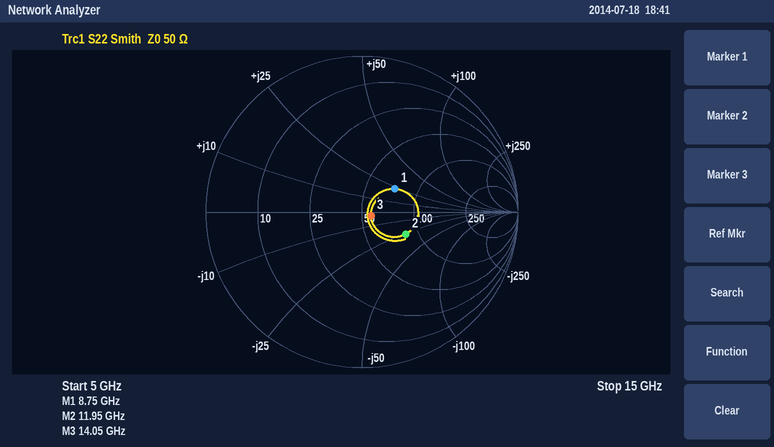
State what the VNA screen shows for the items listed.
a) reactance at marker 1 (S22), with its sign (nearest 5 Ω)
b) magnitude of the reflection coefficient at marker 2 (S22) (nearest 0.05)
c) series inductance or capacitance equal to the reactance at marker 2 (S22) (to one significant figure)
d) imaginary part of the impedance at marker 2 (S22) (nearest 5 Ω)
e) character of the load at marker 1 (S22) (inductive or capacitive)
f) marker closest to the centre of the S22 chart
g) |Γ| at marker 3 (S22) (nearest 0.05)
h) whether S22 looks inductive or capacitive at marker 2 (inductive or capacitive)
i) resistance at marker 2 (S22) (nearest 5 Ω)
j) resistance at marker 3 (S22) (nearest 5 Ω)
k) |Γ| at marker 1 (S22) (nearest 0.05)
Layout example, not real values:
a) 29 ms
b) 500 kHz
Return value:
a) +25 Ω
b) 0.30
c) 500 fF
d) -25 Ω
e) inductive
f) marker 3
g) 0.05
h) capacitive
i) 85 Ω
j) 55 Ω
k) 0.25
